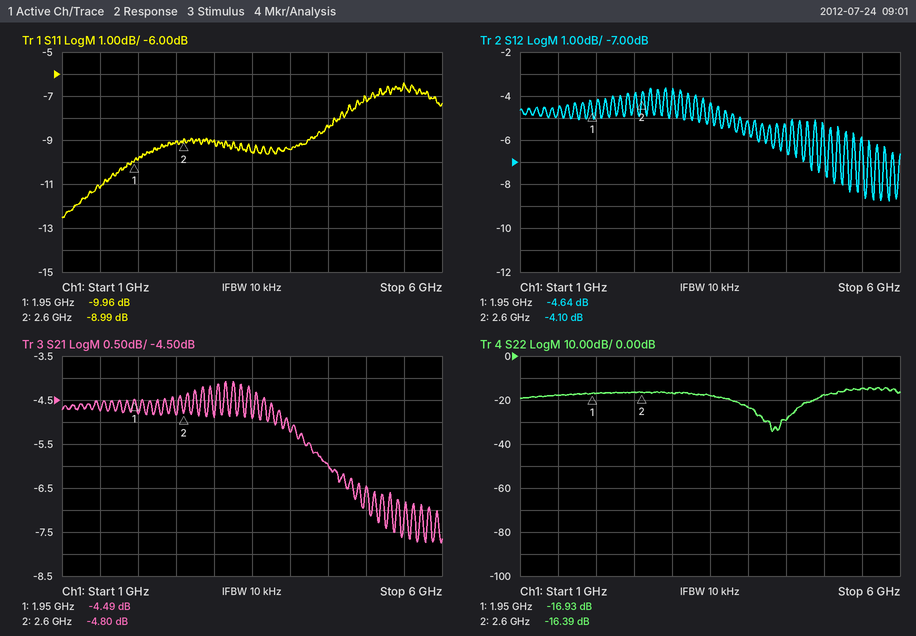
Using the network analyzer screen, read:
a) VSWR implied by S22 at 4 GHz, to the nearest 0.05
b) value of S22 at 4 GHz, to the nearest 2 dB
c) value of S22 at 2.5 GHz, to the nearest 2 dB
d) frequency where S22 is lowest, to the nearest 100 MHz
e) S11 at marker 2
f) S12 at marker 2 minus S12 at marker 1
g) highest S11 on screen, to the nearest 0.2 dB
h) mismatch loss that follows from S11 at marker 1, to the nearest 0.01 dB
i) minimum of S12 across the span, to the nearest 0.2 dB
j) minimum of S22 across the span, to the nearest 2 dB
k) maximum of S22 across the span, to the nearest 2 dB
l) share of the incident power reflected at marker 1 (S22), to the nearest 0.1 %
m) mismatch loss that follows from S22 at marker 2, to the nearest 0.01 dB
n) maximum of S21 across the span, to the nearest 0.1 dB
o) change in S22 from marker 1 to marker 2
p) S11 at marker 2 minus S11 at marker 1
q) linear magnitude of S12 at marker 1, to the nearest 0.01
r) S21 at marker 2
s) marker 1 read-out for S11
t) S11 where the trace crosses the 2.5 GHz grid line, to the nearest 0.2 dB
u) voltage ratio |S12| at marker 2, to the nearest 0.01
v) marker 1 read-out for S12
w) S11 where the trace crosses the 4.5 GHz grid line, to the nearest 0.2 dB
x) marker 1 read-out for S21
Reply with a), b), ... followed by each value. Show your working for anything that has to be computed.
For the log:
a) |Γ| = 10^(-24/20) = 0.0631; VSWR = (1 + 0.0631)/(1 − 0.0631) ≈ 1.13, so 1.15 to the nearest 0.05
b) -24 dB
c) -16 dB
d) 4.3 GHz
e) -8.99 dB
f) -4.1 − (-4.64) = 0.54 dB
g) -6.4 dB
h) −10 log10(1 − 10^(-9.96/10)) ≈ 0.46 dB
i) -8.8 dB
j) -34 dB
k) -14 dB
l) 10^(-16.93/10) ≈ 2.0 %
m) −10 log10(1 − 10^(-16.39/10)) ≈ 0.10 dB
n) -4.1 dB
o) -16.39 − (-16.93) = 0.54 dB
p) -8.99 − (-9.96) = 0.97 dB
q) 10^(-4.64/20) ≈ 0.59
r) -4.80 dB
s) -9.96 dB
t) -9.0 dB
u) 10^(-4.1/20) ≈ 0.62
v) -4.64 dB
w) -8.4 dB
x) -4.49 dB
